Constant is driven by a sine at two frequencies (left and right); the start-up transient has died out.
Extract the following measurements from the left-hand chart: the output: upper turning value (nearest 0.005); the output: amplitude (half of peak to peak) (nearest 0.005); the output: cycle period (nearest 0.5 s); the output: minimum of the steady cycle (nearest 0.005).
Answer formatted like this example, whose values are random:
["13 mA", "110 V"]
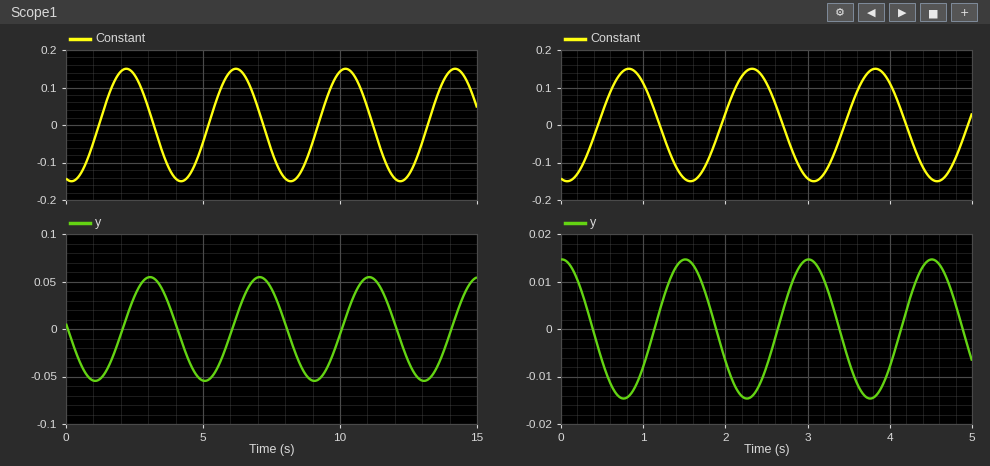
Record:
["0.055", "0.055", "4.0 s", "-0.055"]
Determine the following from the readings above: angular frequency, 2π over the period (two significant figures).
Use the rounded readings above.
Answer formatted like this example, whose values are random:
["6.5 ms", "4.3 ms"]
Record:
["1.6 rad/s"]
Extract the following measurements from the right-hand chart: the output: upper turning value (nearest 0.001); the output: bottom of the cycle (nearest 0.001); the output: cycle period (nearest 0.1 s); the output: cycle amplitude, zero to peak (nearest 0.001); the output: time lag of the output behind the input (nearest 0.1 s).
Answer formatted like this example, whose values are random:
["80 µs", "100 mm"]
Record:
["0.015", "-0.015", "1.5 s", "0.015", "0.7 s"]
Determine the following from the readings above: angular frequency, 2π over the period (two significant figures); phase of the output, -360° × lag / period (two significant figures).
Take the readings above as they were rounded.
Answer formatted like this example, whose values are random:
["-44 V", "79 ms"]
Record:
["4.2 rad/s", "-170°"]
